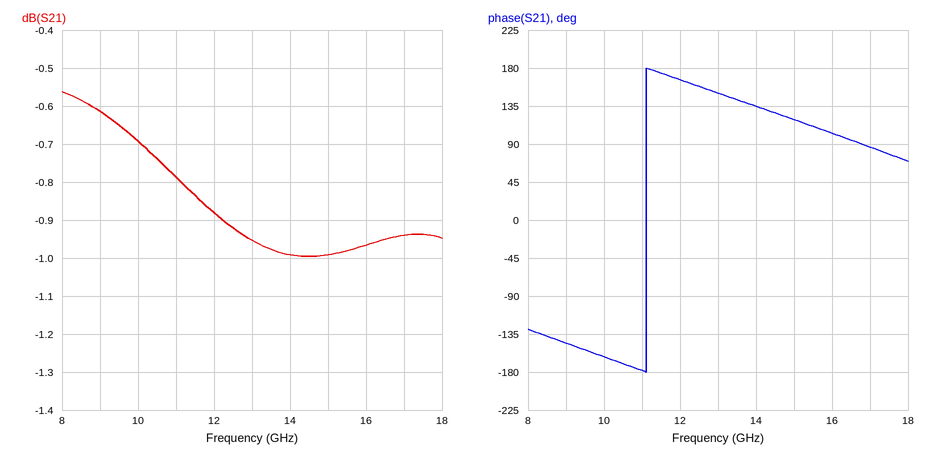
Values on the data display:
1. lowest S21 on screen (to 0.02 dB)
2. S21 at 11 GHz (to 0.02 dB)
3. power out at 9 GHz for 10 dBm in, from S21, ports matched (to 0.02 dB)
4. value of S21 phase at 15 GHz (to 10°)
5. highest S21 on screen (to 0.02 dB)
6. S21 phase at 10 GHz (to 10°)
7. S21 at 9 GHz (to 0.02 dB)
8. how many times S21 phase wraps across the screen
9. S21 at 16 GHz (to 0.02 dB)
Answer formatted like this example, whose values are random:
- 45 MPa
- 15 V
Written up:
- -1.00 dB
- -0.78 dB
- 9.38 dBm
- 120°
- -0.56 dB
- -160°
- -0.62 dB
- 1
- -0.96 dB
